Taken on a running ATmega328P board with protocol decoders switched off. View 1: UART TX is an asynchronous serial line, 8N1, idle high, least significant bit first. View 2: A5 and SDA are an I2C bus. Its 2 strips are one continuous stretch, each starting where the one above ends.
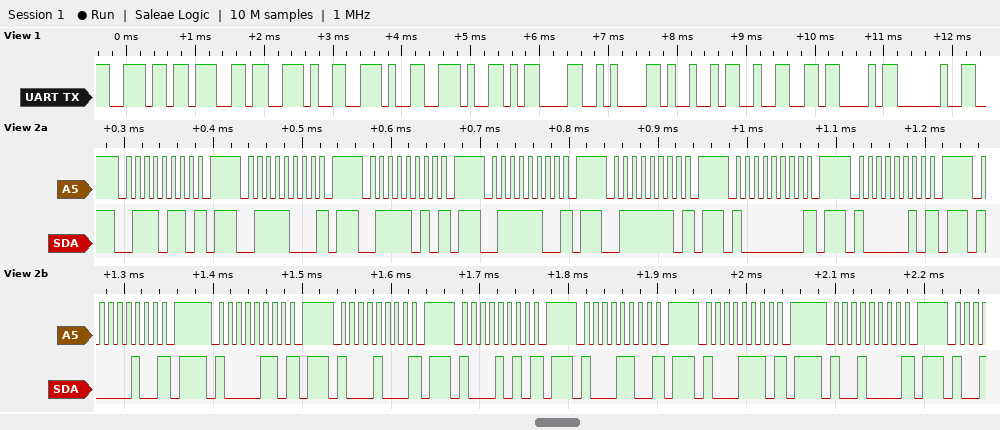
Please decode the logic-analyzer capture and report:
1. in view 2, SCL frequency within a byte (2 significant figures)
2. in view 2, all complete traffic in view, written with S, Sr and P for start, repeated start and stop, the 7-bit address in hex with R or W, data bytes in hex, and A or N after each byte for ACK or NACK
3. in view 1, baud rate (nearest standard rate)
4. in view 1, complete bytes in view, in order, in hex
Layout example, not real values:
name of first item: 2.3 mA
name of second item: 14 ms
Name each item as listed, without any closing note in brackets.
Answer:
in view 2, SCL frequency within a byte: 100 kHz
in view 2, all complete traffic in view, written with S, Sr and P for start, repeated start and stop, the 7-bit address in hex with R or W, data bytes in hex, and A or N after each byte for ACK or NACK: S 3BW N P S 3CW N P S 3DW N P S 3EW N P S 3FW N P S 40W N P S 41W N P S 42W N P S 43W N P S 44W N P S 45W N P S 46W N P S 47W N P S 48W N P
in view 1, baud rate: 9600 baud
in view 1, complete bytes in view, in order, in hex: 0x6E 0x67 0x2E 0x2E 0x2E 0x0D 0x0A 0x49 0x32 0x43 0x20
